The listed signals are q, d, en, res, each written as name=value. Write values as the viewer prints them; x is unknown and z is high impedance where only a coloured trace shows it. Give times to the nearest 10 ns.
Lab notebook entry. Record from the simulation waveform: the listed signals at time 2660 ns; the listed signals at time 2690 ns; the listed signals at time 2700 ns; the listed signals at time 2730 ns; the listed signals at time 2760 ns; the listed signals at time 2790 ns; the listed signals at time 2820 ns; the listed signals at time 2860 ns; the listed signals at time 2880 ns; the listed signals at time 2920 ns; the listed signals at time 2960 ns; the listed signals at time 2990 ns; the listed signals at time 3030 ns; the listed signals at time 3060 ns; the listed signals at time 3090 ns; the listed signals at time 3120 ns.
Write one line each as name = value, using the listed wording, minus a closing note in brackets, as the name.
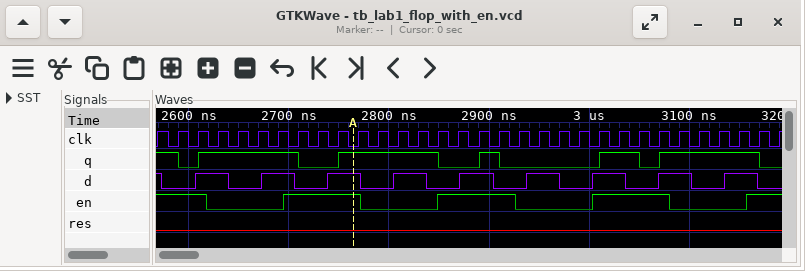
the listed signals at time 2660 ns = q=1, d=0, en=0, res=0
the listed signals at time 2690 ns = q=1, d=1, en=0, res=0
the listed signals at time 2700 ns = q=1, d=1, en=1, res=0
the listed signals at time 2730 ns = q=0, d=0, en=1, res=0
the listed signals at time 2760 ns = q=1, d=1, en=1, res=0
the listed signals at time 2790 ns = q=1, d=0, en=0, res=0
the listed signals at time 2820 ns = q=1, d=1, en=0, res=0
the listed signals at time 2860 ns = q=0, d=0, en=1, res=0
the listed signals at time 2880 ns = q=0, d=1, en=1, res=0
the listed signals at time 2920 ns = q=0, d=0, en=1, res=0
the listed signals at time 2960 ns = q=0, d=1, en=0, res=0
the listed signals at time 2990 ns = q=0, d=0, en=0, res=0
the listed signals at time 3030 ns = q=1, d=1, en=1, res=0
the listed signals at time 3060 ns = q=0, d=0, en=1, res=0
the listed signals at time 3090 ns = q=1, d=1, en=0, res=0
the listed signals at time 3120 ns = q=1, d=0, en=0, res=0
